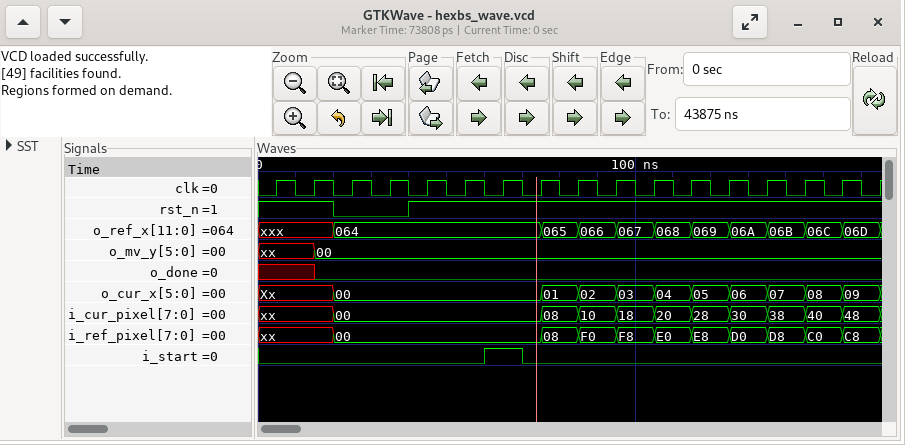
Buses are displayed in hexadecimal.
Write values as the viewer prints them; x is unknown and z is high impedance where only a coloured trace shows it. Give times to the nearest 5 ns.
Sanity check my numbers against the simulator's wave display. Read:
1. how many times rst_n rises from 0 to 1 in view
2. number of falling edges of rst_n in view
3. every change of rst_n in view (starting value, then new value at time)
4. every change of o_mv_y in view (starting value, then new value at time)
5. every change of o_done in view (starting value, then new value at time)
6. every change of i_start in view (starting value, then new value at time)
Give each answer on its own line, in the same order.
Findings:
1
1
1, 0 at 20 ns, 1 at 40 ns
xx, 00 at 15 ns
x, 0 at 15 ns
0, 1 at 60 ns, 0 at 70 ns
